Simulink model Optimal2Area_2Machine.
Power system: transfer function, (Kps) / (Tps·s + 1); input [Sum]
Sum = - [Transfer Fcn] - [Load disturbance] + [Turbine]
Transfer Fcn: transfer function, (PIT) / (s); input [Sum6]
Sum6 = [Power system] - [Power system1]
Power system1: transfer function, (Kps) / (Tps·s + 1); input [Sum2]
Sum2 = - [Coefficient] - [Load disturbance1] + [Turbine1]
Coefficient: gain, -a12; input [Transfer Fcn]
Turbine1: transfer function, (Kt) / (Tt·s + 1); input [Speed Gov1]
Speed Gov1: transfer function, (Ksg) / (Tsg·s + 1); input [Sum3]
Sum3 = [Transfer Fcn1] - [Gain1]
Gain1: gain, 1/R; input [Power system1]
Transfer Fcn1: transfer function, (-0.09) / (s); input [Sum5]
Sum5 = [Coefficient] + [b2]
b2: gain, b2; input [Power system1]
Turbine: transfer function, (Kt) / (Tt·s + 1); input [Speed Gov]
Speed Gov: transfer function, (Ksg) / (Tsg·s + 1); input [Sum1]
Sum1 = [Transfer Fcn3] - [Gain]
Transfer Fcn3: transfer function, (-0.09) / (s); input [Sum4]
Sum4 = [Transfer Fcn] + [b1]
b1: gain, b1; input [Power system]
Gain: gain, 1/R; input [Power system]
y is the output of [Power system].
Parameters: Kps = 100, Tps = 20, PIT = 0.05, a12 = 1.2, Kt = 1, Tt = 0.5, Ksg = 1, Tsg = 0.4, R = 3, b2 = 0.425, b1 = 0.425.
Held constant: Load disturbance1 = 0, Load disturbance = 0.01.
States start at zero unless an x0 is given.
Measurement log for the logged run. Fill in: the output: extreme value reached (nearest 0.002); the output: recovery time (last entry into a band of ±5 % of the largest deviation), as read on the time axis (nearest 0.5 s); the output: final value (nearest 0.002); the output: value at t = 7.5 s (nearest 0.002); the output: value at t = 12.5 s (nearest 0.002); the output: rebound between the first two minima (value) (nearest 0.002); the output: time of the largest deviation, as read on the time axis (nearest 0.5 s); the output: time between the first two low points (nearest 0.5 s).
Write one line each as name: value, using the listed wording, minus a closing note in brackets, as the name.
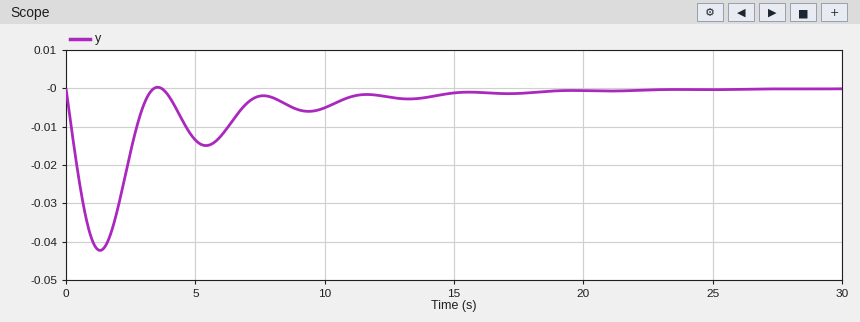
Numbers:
the output: extreme value reached: -0.042
the output: recovery time (last entry into a band of ±5 % of the largest deviation), as read on the time axis: 14.0 s
the output: final value: 0.000
the output: value at t = 7.5 s: -0.002
the output: value at t = 12.5 s: -0.002
the output: rebound between the first two minima (value): 0.000
the output: time of the largest deviation, as read on the time axis: 1.5 s
the output: time between the first two low points: 4.0 s
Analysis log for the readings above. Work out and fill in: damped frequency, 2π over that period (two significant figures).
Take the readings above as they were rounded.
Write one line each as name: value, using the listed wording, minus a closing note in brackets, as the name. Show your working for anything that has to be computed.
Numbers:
damped frequency, 2π over that period: 2π / 4 = 1.6 rad/s
